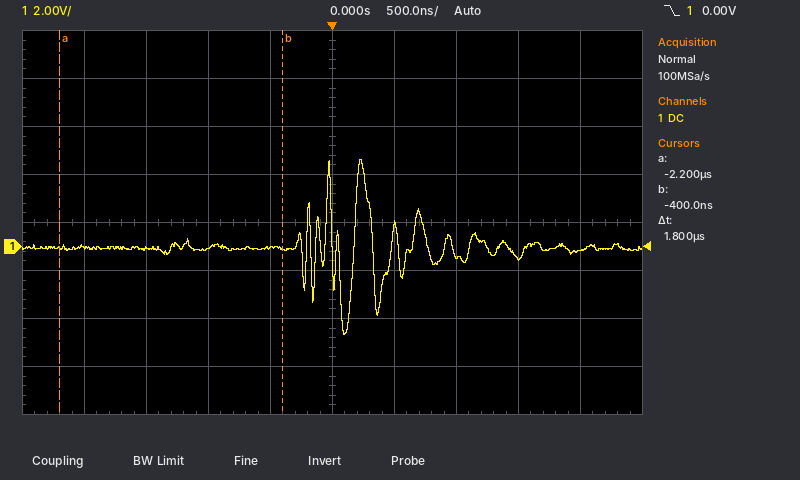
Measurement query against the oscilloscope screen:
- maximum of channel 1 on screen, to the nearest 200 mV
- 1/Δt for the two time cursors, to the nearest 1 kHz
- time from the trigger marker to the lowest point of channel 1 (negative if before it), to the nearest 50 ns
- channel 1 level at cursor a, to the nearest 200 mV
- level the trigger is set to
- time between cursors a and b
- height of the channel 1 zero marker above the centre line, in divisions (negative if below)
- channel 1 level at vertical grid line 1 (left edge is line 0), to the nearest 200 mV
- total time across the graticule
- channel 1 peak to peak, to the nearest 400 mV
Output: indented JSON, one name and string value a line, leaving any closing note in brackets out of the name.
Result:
{
  "maximum of channel 1 on screen, to the nearest 200 mV": "3.6 V",
  "1/Δt for the two time cursors, to the nearest 1 kHz": "556 kHz",
  "time from the trigger marker to the lowest point of channel 1 (negative if before it), to the nearest 50 ns": "+100 ns",
  "channel 1 level at cursor a, to the nearest 200 mV": "0.0 V",
  "level the trigger is set to": "0.00 V",
  "time between cursors a and b": "1.8 µs",
  "height of the channel 1 zero marker above the centre line, in divisions": "-0.5 div",
  "channel 1 level at vertical grid line 1 (left edge is line 0), to the nearest 200 mV": "0.0 V",
  "total time across the graticule": "5 µs",
  "channel 1 peak to peak, to the nearest 400 mV": "7.2 V"
}
